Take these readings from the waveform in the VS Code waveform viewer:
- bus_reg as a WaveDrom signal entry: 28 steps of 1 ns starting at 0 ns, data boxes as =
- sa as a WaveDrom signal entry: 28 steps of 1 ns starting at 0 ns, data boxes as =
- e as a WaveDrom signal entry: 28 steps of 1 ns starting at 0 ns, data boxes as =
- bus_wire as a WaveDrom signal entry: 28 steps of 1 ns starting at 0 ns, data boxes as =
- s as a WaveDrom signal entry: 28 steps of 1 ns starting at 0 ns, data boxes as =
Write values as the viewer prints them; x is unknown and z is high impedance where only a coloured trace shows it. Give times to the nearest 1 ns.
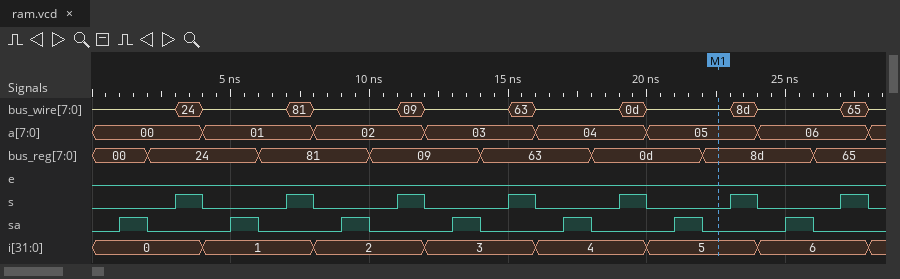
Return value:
{name: 'bus_reg', wave: '=.=...=...=...=...=...=...=.', data: '00 24 81 09 63 0d 8d 65'}
{name: 'sa', wave: '010..10..10..10..10..10..10.'}
{name: 'e', wave: '0...........................'}
{name: 'bus_wire', wave: 'z..=z..=z..=z..=z..=z..=z..=', data: '24 81 09 63 0d 8d 65'}
{name: 's', wave: '0..10..10..10..10..10..10..1'}
